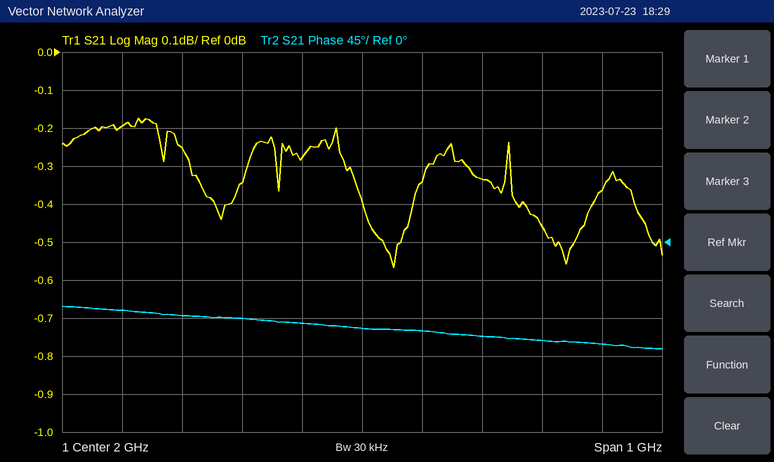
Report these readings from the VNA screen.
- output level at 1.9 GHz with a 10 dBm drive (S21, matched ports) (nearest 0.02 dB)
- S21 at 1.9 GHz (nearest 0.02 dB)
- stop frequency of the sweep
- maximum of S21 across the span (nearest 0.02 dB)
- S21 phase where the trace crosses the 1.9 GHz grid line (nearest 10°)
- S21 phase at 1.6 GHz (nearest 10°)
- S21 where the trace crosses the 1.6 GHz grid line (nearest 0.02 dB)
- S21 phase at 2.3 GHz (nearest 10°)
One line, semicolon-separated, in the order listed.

9.72 dBm; -0.28 dB; 2.5 GHz; -0.18 dB; -100°; -80°; -0.20 dB; -120°
